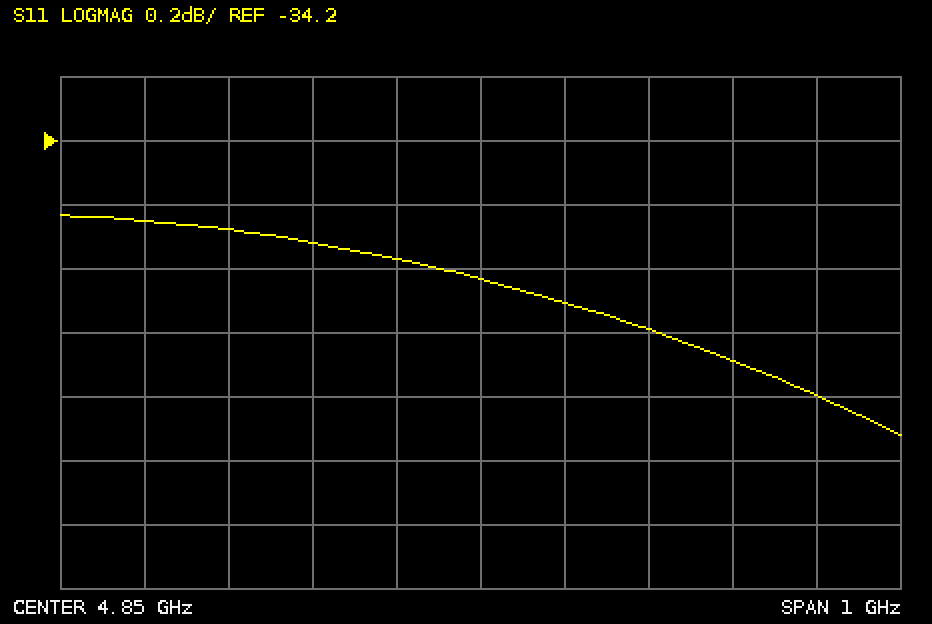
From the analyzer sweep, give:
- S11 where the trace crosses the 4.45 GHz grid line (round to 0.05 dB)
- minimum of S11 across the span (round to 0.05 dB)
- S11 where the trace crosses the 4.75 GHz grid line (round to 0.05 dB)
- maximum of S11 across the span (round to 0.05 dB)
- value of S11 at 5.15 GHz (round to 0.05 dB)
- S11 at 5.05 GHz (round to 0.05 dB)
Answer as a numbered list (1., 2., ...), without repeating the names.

1. -34.45 dB
2. -35.10 dB
3. -34.55 dB
4. -34.45 dB
5. -34.90 dB
6. -34.80 dB
